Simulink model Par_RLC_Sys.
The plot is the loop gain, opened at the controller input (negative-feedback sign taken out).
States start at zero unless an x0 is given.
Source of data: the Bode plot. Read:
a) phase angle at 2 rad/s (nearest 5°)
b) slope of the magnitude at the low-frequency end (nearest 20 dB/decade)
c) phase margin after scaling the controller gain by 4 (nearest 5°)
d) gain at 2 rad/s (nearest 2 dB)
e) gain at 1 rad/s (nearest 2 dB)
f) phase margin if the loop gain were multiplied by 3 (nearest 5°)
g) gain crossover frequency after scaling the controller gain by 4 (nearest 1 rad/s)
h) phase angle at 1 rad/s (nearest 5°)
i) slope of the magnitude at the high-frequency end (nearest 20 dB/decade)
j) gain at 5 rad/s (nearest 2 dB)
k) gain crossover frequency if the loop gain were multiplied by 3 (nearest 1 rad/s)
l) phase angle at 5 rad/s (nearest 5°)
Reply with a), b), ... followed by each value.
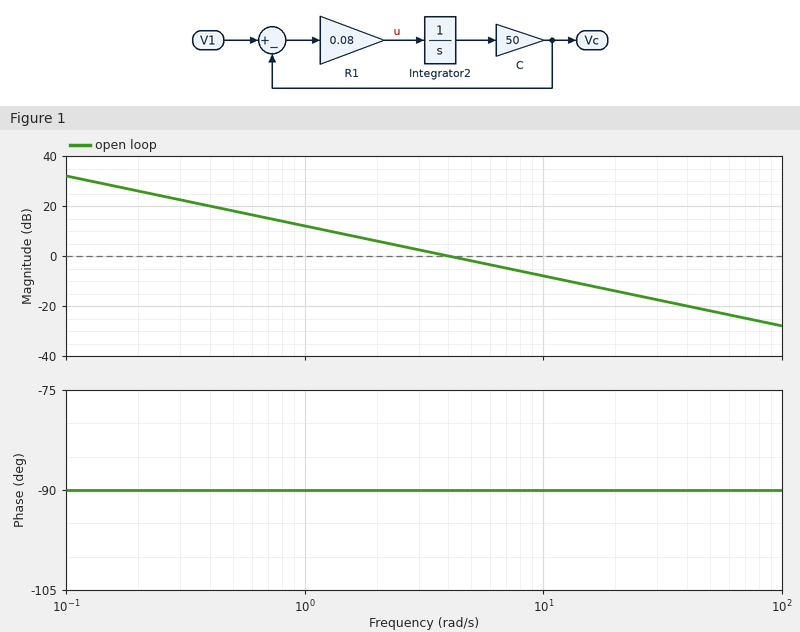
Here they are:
a) -90°
b) -20 dB/decade
c) 90°
d) 6 dB
e) 12 dB
f) 90°
g) 16 rad/s
h) -90°
i) -20 dB/decade
j) -2 dB
k) 12 rad/s
l) -90°
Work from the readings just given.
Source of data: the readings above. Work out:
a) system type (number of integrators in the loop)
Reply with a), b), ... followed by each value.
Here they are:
a) 1
